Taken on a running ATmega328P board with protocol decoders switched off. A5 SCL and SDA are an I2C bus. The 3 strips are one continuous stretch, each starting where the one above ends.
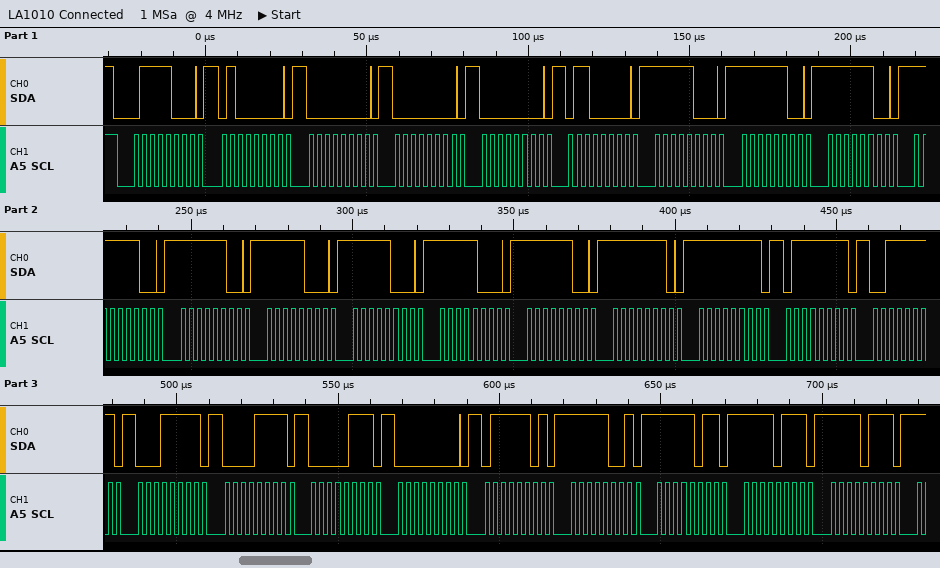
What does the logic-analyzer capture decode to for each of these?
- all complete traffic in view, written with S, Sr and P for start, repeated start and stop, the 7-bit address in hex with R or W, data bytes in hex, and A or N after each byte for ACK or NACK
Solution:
S 3CW A 40 A 00 A 00 A 00 A 60 A F8 A FC A FC A FC A FC A F8 A F8 A F8 A FC A FE A FF A 7F A 3F A 1F A 0F A 07 A 00 A 7D A F9 A FB A F7 A F7 A
